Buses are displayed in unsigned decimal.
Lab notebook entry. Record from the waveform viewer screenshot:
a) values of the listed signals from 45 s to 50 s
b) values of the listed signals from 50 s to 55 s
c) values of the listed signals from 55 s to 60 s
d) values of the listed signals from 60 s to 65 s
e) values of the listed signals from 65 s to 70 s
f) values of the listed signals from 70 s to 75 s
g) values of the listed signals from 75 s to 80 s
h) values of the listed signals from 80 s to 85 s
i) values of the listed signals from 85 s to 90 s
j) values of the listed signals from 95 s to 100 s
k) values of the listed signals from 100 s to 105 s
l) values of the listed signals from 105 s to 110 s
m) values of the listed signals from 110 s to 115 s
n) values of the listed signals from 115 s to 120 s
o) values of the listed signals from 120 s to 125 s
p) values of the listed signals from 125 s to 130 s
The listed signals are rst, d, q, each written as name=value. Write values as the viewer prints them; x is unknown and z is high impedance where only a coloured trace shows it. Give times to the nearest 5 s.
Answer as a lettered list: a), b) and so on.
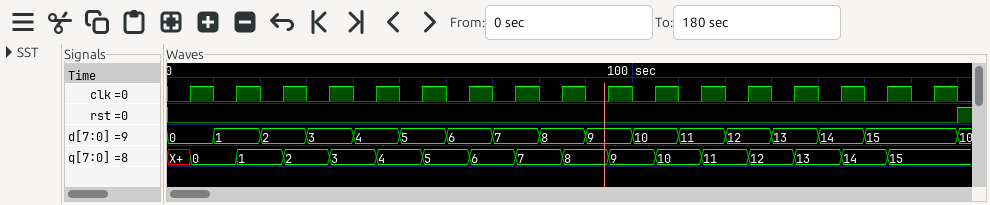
a) rst=0, d=4, q=4
b) rst=0, d=5, q=4
c) rst=0, d=5, q=5
d) rst=0, d=6, q=5
e) rst=0, d=6, q=6
f) rst=0, d=7, q=6
g) rst=0, d=7, q=7
h) rst=0, d=8, q=7
i) rst=0, d=8, q=8
j) rst=0, d=9, q=9
k) rst=0, d=10, q=9
l) rst=0, d=10, q=10
m) rst=0, d=11, q=10
n) rst=0, d=11, q=11
o) rst=0, d=12, q=11
p) rst=0, d=12, q=12
